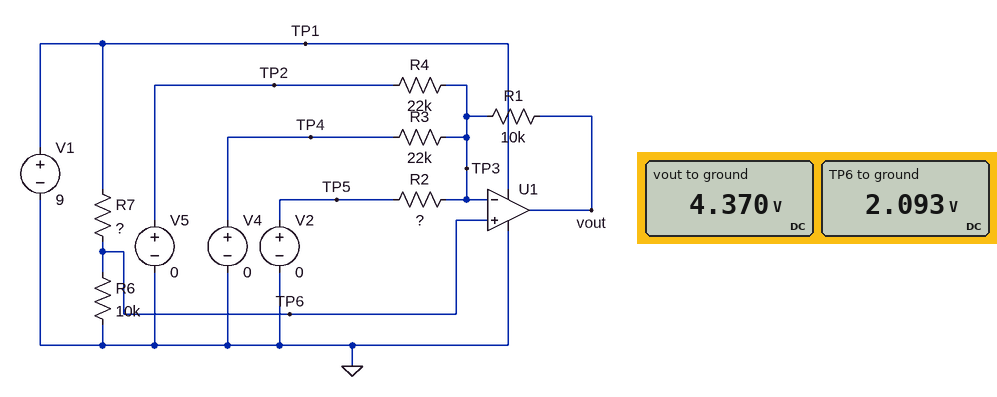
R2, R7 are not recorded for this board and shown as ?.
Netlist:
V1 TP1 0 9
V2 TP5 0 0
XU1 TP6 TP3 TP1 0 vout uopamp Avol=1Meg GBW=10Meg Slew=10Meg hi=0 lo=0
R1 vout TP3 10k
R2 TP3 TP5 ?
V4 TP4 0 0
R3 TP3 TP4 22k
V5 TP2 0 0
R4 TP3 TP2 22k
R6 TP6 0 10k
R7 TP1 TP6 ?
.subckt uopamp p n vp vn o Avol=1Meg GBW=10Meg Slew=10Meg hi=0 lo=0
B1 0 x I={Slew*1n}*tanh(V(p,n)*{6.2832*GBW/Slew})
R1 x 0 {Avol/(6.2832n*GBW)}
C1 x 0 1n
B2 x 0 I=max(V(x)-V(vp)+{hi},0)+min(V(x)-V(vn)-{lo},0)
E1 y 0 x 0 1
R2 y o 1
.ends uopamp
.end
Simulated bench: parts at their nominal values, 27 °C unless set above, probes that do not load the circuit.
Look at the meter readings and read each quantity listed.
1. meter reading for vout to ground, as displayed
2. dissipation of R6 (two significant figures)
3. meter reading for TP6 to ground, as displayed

4.370 V
440 µW
2.093 V
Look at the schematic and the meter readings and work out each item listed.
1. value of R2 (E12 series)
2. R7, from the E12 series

56 kΩ
33 kΩ
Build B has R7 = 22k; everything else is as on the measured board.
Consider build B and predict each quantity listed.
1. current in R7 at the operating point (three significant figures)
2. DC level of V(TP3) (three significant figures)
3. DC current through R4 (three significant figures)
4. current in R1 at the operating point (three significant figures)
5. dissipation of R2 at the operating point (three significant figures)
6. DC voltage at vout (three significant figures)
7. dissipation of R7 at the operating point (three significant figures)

281 µA
2.81 V
128 µA
306 µA
141 µW
5.87 V
1.74 mW
